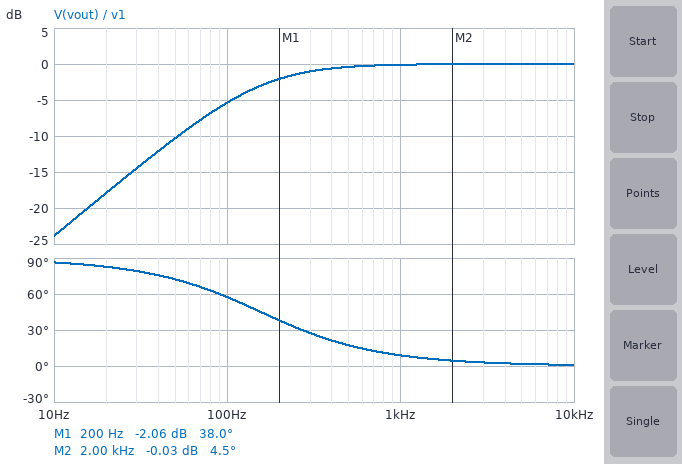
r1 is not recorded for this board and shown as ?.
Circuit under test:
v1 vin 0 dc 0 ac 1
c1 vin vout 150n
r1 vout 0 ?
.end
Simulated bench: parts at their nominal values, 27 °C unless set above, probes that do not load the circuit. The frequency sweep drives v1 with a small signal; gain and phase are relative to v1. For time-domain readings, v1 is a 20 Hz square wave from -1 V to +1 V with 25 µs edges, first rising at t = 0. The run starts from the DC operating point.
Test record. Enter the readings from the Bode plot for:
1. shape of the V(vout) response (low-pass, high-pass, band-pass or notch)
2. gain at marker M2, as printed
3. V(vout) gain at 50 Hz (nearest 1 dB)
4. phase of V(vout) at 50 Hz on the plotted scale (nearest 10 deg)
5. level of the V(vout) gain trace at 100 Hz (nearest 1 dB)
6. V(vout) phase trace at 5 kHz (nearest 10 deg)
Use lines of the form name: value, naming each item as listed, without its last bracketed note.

shape of the V(vout) response: high-pass
gain at marker M2, as printed: -0.03 dB
V(vout) gain at 50 Hz: -10 dB
phase of V(vout) at 50 Hz on the plotted scale: 70 deg
level of the V(vout) gain trace at 100 Hz: -5 dB
V(vout) phase trace at 5 kHz: 0 deg
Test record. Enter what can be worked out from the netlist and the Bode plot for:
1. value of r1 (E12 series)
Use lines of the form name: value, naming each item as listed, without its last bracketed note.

value of r1: 6.8 kΩ
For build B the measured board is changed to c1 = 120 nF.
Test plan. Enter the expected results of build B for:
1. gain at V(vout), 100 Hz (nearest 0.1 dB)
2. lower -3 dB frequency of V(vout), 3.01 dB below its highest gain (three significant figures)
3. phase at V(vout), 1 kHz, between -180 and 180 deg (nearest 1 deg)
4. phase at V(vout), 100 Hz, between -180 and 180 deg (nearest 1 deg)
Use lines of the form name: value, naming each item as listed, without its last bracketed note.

gain at V(vout), 100 Hz: -6.8 dB
lower -3 dB frequency of V(vout), 3.01 dB below its highest gain: 195 Hz
phase at V(vout), 1 kHz, between -180 and 180 deg: 11 deg
phase at V(vout), 100 Hz, between -180 and 180 deg: 63 deg
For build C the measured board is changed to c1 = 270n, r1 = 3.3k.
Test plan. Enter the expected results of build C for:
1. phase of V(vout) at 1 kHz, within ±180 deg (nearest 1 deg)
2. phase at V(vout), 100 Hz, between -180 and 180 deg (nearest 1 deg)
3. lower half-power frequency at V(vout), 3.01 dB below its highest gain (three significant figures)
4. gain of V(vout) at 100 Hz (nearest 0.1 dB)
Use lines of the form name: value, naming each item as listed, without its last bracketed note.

phase of V(vout) at 1 kHz, within ±180 deg: 10 deg
phase at V(vout), 100 Hz, between -180 and 180 deg: 61 deg
lower half-power frequency at V(vout), 3.01 dB below its highest gain: 179 Hz
gain of V(vout) at 100 Hz: -6.2 dB
